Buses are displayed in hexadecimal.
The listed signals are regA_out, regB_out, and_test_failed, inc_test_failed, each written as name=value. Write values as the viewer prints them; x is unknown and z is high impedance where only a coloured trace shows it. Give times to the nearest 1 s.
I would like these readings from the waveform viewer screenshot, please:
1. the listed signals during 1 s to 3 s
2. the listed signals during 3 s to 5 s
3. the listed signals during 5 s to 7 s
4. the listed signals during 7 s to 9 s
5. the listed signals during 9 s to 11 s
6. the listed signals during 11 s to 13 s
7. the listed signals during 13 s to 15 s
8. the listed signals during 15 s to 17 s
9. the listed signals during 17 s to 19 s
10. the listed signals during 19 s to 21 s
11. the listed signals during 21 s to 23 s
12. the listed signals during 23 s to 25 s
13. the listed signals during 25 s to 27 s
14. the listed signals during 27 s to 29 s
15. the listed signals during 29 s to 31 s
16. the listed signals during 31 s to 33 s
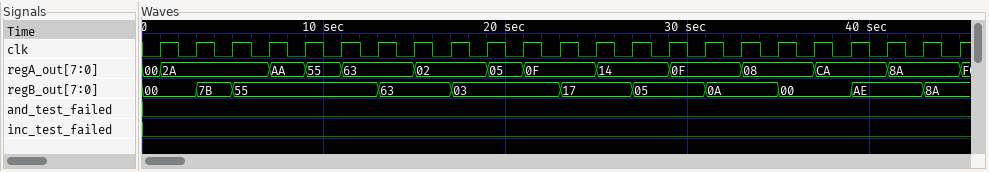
regA_out=2A, regB_out=00, and_test_failed=0, inc_test_failed=0
regA_out=2A, regB_out=7B, and_test_failed=0, inc_test_failed=0
regA_out=2A, regB_out=55, and_test_failed=0, inc_test_failed=0
regA_out=AA, regB_out=55, and_test_failed=0, inc_test_failed=0
regA_out=55, regB_out=55, and_test_failed=0, inc_test_failed=0
regA_out=63, regB_out=55, and_test_failed=0, inc_test_failed=0
regA_out=63, regB_out=63, and_test_failed=0, inc_test_failed=0
regA_out=02, regB_out=63, and_test_failed=0, inc_test_failed=0
regA_out=02, regB_out=03, and_test_failed=0, inc_test_failed=0
regA_out=05, regB_out=03, and_test_failed=0, inc_test_failed=0
regA_out=0F, regB_out=03, and_test_failed=0, inc_test_failed=0
regA_out=0F, regB_out=17, and_test_failed=0, inc_test_failed=0
regA_out=14, regB_out=17, and_test_failed=0, inc_test_failed=0
regA_out=14, regB_out=05, and_test_failed=0, inc_test_failed=0
regA_out=0F, regB_out=05, and_test_failed=0, inc_test_failed=0
regA_out=0F, regB_out=0A, and_test_failed=0, inc_test_failed=0
